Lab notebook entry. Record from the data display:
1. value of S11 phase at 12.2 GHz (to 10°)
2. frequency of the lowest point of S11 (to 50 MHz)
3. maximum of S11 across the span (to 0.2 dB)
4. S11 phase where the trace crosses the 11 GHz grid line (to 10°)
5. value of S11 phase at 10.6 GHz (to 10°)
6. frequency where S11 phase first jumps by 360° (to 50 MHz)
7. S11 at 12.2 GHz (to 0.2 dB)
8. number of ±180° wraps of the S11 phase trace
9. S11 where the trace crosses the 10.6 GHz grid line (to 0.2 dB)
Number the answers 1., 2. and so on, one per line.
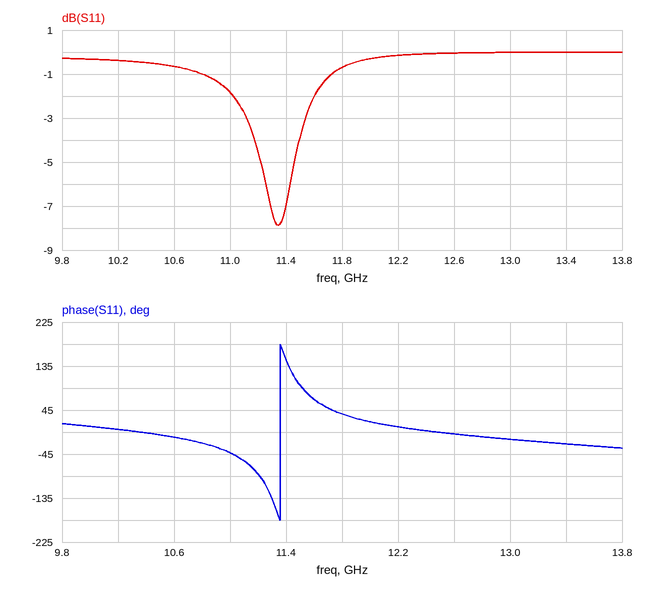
1. 10°
2. 11.35 GHz
3. 0.0 dB
4. -40°
5. -10°
6. 11.35 GHz
7. -0.2 dB
8. 1
9. -0.6 dB
